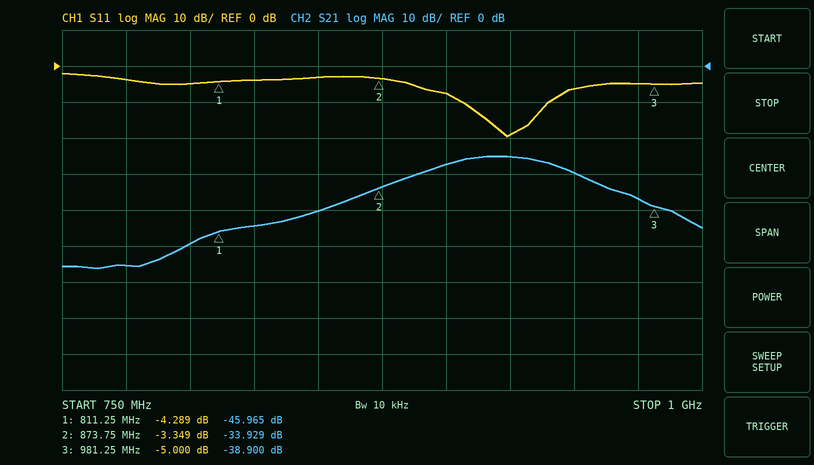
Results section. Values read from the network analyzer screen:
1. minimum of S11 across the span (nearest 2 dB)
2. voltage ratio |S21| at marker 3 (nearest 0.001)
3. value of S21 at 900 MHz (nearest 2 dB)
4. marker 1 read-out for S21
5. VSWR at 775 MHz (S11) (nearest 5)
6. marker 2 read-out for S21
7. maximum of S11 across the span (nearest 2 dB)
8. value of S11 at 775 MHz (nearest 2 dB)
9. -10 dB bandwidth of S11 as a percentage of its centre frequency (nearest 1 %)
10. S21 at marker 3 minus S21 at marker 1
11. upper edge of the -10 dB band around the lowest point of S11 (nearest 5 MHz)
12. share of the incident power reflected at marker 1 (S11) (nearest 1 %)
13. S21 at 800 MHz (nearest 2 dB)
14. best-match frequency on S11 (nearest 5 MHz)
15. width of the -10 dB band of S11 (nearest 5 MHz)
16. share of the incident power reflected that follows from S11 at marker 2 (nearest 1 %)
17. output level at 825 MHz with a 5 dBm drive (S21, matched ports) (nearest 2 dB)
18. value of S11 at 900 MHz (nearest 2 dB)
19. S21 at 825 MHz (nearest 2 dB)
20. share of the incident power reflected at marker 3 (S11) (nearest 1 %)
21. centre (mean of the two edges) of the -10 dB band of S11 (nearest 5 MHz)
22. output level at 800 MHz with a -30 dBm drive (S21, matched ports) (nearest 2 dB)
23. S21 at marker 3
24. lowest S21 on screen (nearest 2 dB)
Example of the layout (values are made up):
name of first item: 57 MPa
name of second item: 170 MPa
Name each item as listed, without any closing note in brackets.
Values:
minimum of S11 across the span: -20 dB
voltage ratio |S21| at marker 3: 0.011
value of S21 at 900 MHz: -28 dB
marker 1 read-out for S21: -45.965 dB
VSWR at 775 MHz (S11): 5
marker 2 read-out for S21: -33.929 dB
maximum of S11 across the span: -2 dB
value of S11 at 775 MHz: -4 dB
-10 dB bandwidth of S11 as a percentage of its centre frequency: 4 %
S21 at marker 3 minus S21 at marker 1: 7.065 dB
upper edge of the -10 dB band around the lowest point of S11: 940 MHz
share of the incident power reflected at marker 1 (S11): 37 %
S21 at 800 MHz: -50 dB
best-match frequency on S11: 925 MHz
width of the -10 dB band of S11: 35 MHz
share of the incident power reflected that follows from S11 at marker 2: 46 %
output level at 825 MHz with a 5 dBm drive (S21, matched ports): -40 dBm
value of S11 at 900 MHz: -8 dB
S21 at 825 MHz: -44 dB
share of the incident power reflected at marker 3 (S11): 32 %
centre (mean of the two edges) of the -10 dB band of S11: 925 MHz
output level at 800 MHz with a -30 dBm drive (S21, matched ports): -80 dBm
S21 at marker 3: -38.900 dB
lowest S21 on screen: -56 dB
